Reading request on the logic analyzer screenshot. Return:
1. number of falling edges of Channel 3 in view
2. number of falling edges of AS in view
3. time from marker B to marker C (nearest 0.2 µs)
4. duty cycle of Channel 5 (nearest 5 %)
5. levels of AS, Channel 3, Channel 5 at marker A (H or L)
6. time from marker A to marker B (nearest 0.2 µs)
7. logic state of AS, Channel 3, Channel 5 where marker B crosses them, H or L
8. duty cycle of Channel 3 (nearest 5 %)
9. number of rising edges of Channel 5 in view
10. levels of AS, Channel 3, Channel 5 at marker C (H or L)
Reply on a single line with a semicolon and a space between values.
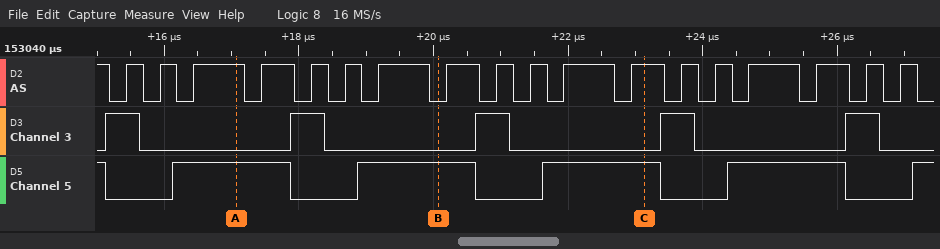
5; 19; 3 µs; 65 %; AS=H, Channel 3=L, Channel 5=H; 3 µs; AS=L, Channel 3=L, Channel 5=H; 20 %; 5; AS=H, Channel 3=L, Channel 5=H
